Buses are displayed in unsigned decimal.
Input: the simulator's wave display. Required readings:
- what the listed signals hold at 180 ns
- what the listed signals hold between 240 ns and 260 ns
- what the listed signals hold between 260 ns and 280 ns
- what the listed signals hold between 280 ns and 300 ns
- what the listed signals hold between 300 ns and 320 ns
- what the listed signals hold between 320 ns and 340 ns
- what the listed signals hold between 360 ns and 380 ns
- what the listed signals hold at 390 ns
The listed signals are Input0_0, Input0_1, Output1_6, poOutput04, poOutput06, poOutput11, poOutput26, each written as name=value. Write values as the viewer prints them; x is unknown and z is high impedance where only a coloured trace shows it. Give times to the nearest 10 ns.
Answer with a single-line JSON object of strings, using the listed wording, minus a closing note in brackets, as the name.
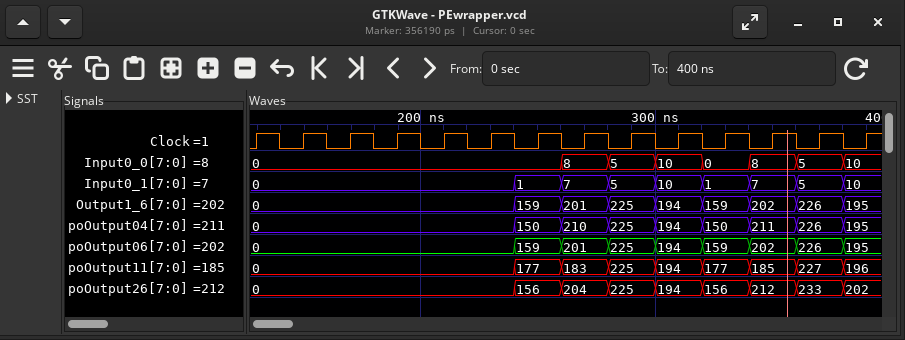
{"what the listed signals hold at 180 ns": "Input0_0=0, Input0_1=0, Output1_6=0, poOutput04=0, poOutput06=0, poOutput11=0, poOutput26=0", "what the listed signals hold between 240 ns and 260 ns": "Input0_0=0, Input0_1=1, Output1_6=159, poOutput04=150, poOutput06=159, poOutput11=177, poOutput26=156", "what the listed signals hold between 260 ns and 280 ns": "Input0_0=8, Input0_1=7, Output1_6=201, poOutput04=210, poOutput06=201, poOutput11=183, poOutput26=204", "what the listed signals hold between 280 ns and 300 ns": "Input0_0=5, Input0_1=5, Output1_6=225, poOutput04=225, poOutput06=225, poOutput11=225, poOutput26=225", "what the listed signals hold between 300 ns and 320 ns": "Input0_0=10, Input0_1=10, Output1_6=194, poOutput04=194, poOutput06=194, poOutput11=194, poOutput26=194", "what the listed signals hold between 320 ns and 340 ns": "Input0_0=0, Input0_1=1, Output1_6=159, poOutput04=150, poOutput06=159, poOutput11=177, poOutput26=156", "what the listed signals hold between 360 ns and 380 ns": "Input0_0=5, Input0_1=5, Output1_6=226, poOutput04=226, poOutput06=226, poOutput11=227, poOutput26=233", "what the listed signals hold at 390 ns": "Input0_0=10, Input0_1=10, Output1_6=195, poOutput04=195, poOutput06=195, poOutput11=196, poOutput26=202"}
